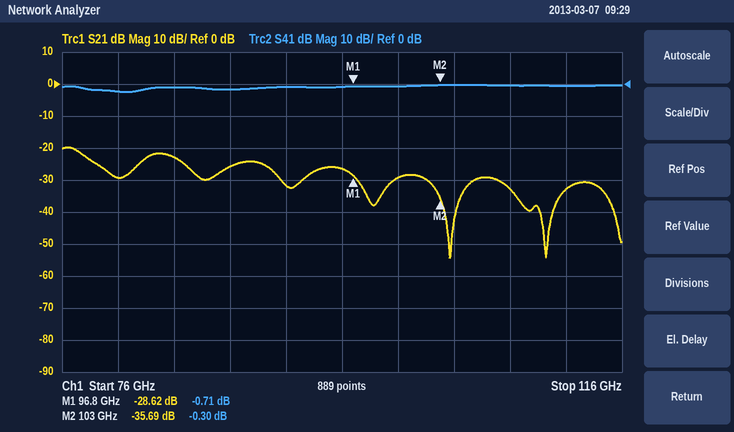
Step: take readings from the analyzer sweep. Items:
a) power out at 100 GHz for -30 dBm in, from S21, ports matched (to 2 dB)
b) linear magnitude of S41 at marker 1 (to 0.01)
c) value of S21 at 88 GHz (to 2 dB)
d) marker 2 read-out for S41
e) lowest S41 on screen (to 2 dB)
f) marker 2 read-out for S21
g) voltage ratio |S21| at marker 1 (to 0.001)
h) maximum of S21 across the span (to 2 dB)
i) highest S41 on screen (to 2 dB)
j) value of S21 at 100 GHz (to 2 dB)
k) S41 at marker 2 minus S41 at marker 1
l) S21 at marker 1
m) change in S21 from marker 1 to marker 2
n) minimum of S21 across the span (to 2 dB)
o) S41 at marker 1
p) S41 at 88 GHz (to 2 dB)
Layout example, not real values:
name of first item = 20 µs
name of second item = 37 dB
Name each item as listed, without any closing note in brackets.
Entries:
power out at 100 GHz for -30 dBm in, from S21, ports matched = -60 dBm
linear magnitude of S41 at marker 1 = 0.92
value of S21 at 88 GHz = -26 dB
marker 2 read-out for S41 = -0.30 dB
lowest S41 on screen = -2 dB
marker 2 read-out for S21 = -35.69 dB
voltage ratio |S21| at marker 1 = 0.037
maximum of S21 across the span = -20 dB
highest S41 on screen = 0 dB
value of S21 at 100 GHz = -30 dB
S41 at marker 2 minus S41 at marker 1 = 0.41 dB
S21 at marker 1 = -28.62 dB
change in S21 from marker 1 to marker 2 = -7.07 dB
minimum of S21 across the span = -54 dB
S41 at marker 1 = -0.71 dB
S41 at 88 GHz = -2 dB
